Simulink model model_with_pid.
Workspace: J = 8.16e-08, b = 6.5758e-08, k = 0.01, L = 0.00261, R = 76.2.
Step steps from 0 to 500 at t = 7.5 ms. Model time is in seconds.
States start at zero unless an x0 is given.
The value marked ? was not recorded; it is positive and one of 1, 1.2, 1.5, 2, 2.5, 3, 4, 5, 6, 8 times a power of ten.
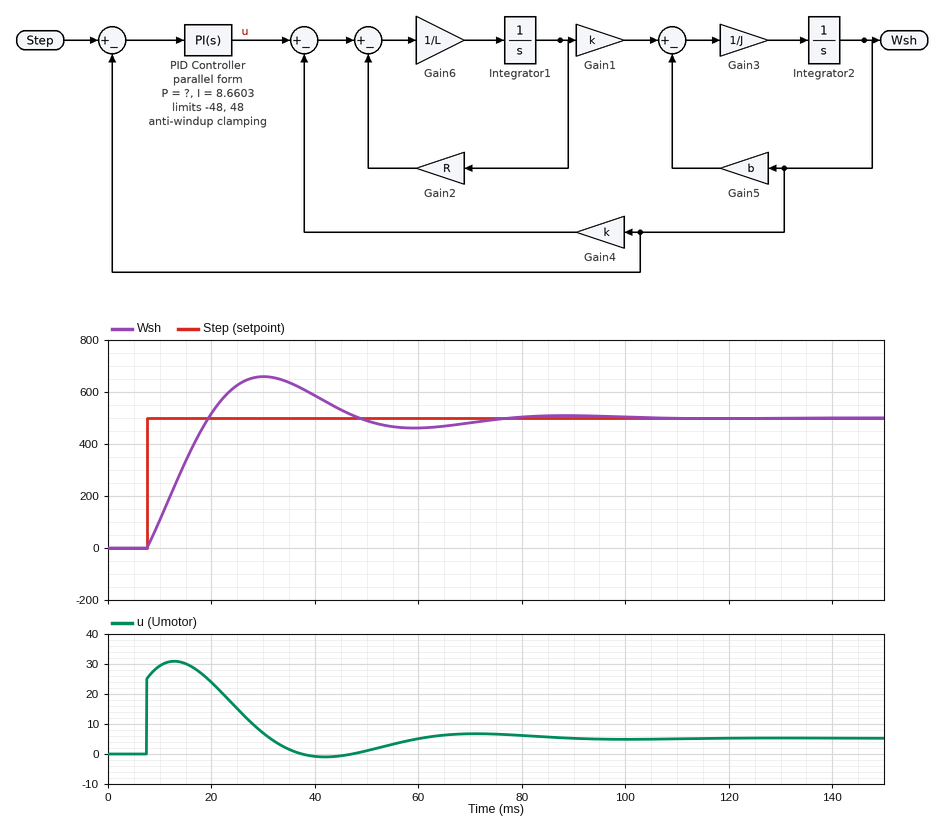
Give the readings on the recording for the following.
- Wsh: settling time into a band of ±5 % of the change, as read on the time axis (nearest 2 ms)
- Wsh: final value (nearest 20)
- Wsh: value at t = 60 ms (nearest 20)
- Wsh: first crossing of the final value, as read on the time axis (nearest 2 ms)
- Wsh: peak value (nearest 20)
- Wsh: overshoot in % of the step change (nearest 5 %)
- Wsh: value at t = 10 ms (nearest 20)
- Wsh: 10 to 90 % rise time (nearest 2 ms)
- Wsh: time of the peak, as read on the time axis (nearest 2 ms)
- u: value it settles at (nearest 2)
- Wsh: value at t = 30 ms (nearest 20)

68 ms
500
460
20 ms
660
30 %
100
10 ms
30 ms
6
660
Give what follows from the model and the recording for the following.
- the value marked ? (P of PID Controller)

0.05
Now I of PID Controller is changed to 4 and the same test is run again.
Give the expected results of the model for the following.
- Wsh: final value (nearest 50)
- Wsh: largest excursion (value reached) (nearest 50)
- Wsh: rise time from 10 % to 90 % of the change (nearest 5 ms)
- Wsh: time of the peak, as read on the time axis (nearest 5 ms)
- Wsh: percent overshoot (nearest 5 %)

500
600
15 ms
40 ms
20 %
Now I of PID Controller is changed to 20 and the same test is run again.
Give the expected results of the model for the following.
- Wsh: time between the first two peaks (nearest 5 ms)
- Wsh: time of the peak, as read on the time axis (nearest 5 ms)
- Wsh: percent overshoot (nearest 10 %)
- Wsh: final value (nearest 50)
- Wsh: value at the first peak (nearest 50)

35 ms
25 ms
50 %
500
750
